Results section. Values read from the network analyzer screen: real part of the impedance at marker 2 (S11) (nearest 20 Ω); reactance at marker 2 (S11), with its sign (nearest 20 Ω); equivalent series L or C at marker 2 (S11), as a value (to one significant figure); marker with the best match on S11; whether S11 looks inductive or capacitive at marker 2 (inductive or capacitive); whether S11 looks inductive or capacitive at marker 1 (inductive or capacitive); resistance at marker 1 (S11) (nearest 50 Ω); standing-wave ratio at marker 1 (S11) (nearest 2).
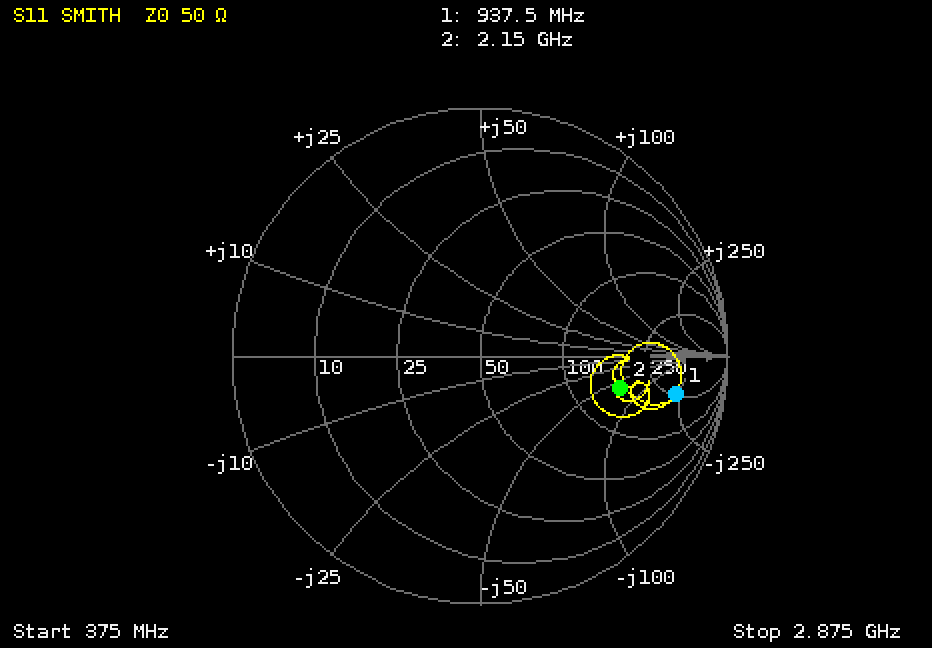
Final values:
160 Ω
-60 Ω
1 pF
marker 2
capacitive
capacitive
250 Ω
10
